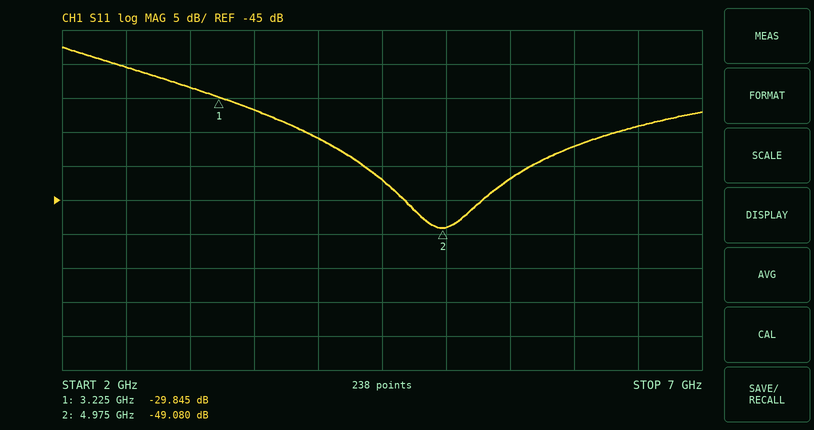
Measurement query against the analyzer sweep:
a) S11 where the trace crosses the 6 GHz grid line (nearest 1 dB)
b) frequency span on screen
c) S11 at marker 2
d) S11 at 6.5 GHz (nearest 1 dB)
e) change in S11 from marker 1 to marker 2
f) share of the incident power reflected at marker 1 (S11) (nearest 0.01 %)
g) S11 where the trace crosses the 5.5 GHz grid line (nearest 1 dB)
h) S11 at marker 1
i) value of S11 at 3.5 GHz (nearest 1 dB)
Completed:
-37 dB
5 GHz
-49.080 dB
-34 dB
-19.235 dB
0.10 %
-42 dB
-29.845 dB
-32 dB
